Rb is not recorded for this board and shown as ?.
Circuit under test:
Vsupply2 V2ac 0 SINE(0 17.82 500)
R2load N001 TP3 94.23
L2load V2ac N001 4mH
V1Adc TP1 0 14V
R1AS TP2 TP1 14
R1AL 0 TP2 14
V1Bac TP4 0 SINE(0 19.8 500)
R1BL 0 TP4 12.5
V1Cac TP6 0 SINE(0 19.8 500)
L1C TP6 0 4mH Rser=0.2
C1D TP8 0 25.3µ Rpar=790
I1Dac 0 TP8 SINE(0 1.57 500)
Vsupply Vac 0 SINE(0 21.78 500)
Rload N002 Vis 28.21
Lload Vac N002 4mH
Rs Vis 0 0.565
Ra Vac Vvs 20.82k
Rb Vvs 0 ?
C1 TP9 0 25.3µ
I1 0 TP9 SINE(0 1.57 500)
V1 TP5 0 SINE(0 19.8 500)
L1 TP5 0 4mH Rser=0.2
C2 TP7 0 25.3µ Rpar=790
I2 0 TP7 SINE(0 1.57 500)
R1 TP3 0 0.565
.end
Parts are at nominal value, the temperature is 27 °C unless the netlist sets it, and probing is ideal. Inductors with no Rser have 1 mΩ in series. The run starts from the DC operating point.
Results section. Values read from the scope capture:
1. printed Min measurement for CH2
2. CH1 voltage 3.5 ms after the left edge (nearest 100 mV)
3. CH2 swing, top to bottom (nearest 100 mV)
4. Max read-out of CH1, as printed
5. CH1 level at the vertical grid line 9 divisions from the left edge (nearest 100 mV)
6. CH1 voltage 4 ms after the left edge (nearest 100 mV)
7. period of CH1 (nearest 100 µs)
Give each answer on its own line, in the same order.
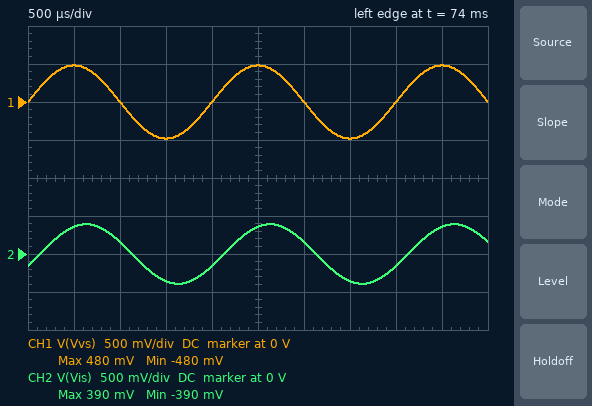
-390 mV
-500 mV
800 mV
480 mV
500 mV
0 V
2.0 ms
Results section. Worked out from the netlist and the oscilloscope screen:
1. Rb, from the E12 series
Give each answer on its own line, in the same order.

470 Ω
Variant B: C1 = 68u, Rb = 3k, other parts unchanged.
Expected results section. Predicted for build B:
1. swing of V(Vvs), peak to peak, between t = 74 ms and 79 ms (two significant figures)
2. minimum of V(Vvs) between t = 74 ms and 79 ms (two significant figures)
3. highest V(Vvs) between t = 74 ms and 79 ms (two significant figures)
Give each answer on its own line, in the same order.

5.5 V
-2.7 V
2.7 V
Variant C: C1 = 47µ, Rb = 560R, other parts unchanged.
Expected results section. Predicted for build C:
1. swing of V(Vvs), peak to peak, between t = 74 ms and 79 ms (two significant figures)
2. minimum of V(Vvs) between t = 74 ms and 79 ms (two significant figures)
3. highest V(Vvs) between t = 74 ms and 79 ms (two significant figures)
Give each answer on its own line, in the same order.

1.1 V
-570 mV
570 mV
